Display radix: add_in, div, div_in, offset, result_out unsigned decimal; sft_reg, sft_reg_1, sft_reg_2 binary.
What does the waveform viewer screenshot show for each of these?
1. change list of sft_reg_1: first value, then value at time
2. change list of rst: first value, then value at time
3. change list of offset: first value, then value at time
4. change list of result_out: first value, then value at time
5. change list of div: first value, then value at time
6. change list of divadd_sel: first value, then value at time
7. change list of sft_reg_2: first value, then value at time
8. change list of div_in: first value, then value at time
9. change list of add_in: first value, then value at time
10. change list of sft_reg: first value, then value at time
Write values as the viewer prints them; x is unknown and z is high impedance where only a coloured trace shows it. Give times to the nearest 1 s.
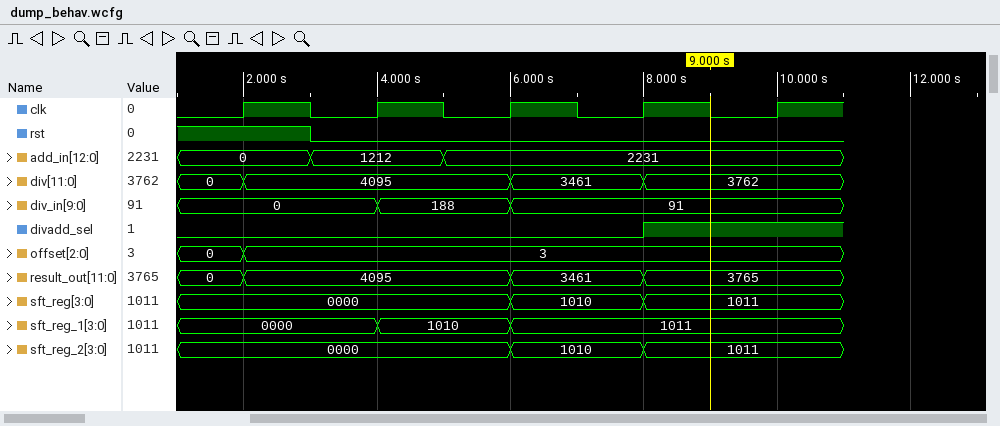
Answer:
0000, 1010 at 4 s, 1011 at 6 s
1, 0 at 3 s
0, 3 at 2 s
0, 4095 at 2 s, 3461 at 6 s, 3765 at 8 s
0, 4095 at 2 s, 3461 at 6 s, 3762 at 8 s
0, 1 at 8 s
0000, 1010 at 6 s, 1011 at 8 s
0, 188 at 4 s, 91 at 6 s
0, 1212 at 3 s, 2231 at 5 s
0000, 1010 at 6 s, 1011 at 8 s
